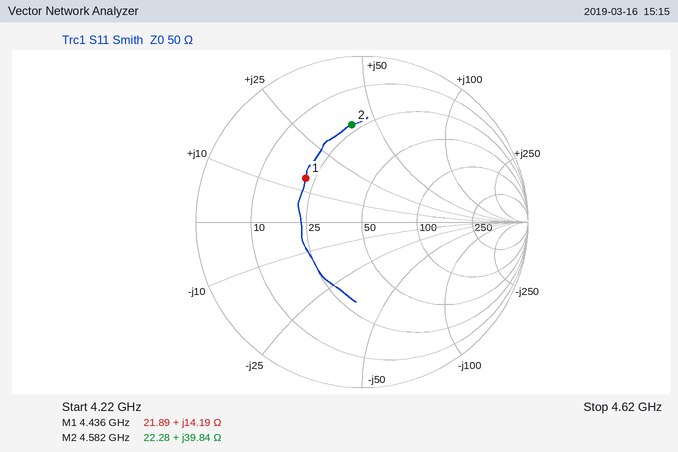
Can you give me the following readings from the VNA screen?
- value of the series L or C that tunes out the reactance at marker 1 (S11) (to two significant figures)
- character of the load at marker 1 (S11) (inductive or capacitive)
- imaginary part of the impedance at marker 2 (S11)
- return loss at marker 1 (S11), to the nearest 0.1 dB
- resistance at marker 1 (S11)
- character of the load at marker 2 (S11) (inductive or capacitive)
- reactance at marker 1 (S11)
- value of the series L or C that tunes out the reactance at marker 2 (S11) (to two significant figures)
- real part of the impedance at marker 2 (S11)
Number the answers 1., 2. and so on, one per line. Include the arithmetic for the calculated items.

1. C = 1/(2π × 4.436 GHz × 14.19 Ω) ≈ 2.5 pF
2. inductive
3. +39.84 Ω
4. 7.3 dB
5. 21.89 Ω
6. inductive
7. +14.19 Ω
8. C = 1/(2π × 4.582 GHz × 39.84 Ω) ≈ 872 fF, so 870 fF to two significant figures
9. 22.28 Ω
